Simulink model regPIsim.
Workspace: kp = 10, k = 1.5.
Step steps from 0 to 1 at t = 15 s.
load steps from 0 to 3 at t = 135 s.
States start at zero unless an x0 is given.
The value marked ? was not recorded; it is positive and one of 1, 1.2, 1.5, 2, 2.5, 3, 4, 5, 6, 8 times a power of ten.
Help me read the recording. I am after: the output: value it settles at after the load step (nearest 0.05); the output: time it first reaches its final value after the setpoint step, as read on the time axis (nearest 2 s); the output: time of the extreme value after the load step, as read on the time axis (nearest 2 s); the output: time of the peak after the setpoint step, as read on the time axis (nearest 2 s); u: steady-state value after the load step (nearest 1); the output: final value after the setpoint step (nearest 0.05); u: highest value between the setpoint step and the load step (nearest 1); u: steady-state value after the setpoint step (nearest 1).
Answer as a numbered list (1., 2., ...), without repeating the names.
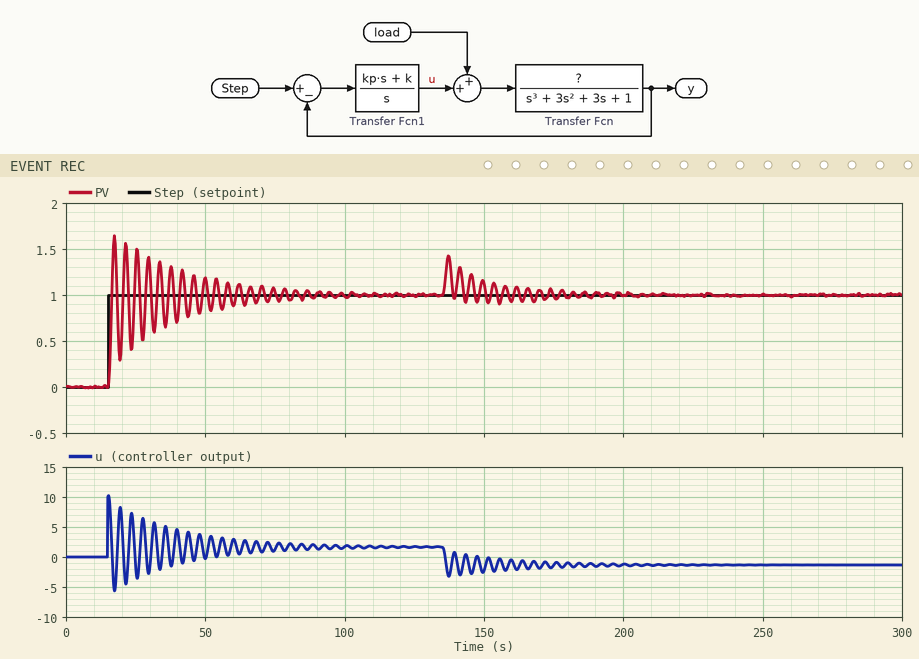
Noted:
1. 1.00
2. 16 s
3. 138 s
4. 18 s
5. -1
6. 1.00
7. 10
8. 2
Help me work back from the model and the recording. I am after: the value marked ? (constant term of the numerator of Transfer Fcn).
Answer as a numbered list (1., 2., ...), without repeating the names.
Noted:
1. 0.6
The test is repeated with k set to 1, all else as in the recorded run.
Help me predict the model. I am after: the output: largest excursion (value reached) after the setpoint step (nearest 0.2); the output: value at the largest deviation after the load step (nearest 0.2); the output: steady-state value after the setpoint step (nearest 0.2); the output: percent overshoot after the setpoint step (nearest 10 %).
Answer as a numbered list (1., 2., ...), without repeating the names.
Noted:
1. 1.6
2. 1.4
3. 1.0
4. 60 %
